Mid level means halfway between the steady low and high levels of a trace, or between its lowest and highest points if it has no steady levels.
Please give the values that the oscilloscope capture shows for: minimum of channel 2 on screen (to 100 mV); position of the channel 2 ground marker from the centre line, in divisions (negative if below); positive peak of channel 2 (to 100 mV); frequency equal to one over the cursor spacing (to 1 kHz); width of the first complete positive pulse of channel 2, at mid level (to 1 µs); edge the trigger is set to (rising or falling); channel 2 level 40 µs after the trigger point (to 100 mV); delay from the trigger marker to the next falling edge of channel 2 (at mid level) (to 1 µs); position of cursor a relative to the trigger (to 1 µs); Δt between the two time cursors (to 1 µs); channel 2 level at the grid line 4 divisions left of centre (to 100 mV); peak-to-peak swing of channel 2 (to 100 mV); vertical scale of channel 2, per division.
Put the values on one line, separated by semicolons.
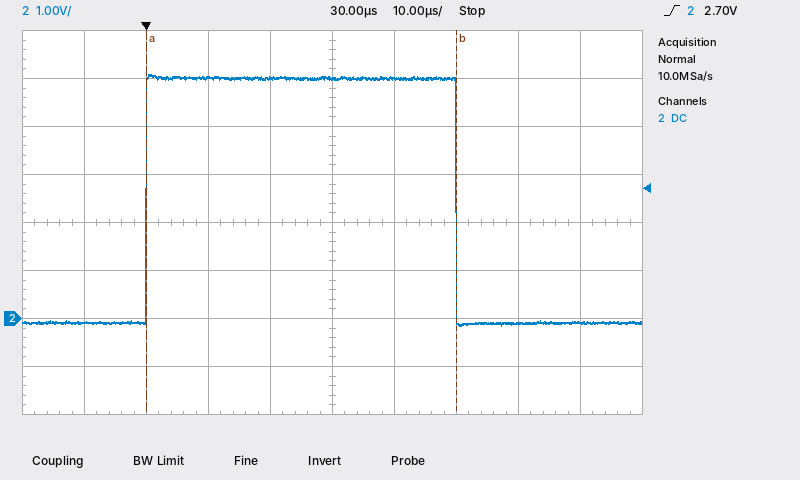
-100 mV; -2.0 div; 5.1 V; 20 kHz; 50 µs; rising; 5.0 V; 50 µs; 0 µs; 50 µs; -100 mV; 5.2 V; 1 V
